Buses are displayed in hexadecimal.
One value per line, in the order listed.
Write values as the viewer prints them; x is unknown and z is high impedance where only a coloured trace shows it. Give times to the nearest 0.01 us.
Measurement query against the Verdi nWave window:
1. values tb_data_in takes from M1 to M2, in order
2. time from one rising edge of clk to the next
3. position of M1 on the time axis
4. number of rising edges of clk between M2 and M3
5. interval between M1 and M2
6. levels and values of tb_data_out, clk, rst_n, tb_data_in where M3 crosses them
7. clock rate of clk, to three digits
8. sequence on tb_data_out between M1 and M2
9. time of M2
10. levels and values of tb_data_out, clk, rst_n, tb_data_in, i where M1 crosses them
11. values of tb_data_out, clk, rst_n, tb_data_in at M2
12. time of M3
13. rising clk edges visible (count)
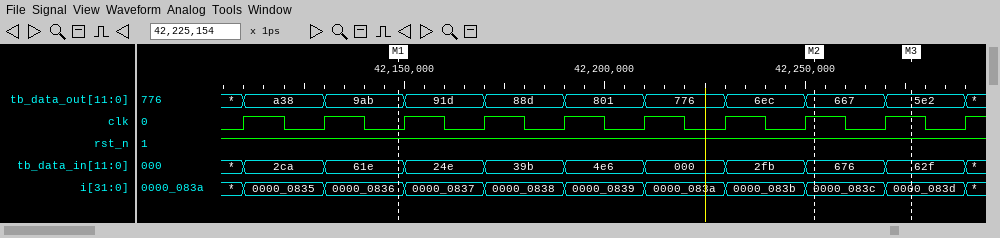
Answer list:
61e, 24e, 39b, 4e6, 000, 2fb, 676
0.02 us
42.15 us
1
0.1 us
tb_data_out=5e2, clk=1, rst_n=1, tb_data_in=62f
50.0 MHz
9ab, 91d, 88d, 801, 776, 6ec, 667
42.25 us
tb_data_out=9ab, clk=0, rst_n=1, tb_data_in=61e, i=0000_0836
tb_data_out=667, clk=1, rst_n=1, tb_data_in=676
42.28 us
10
